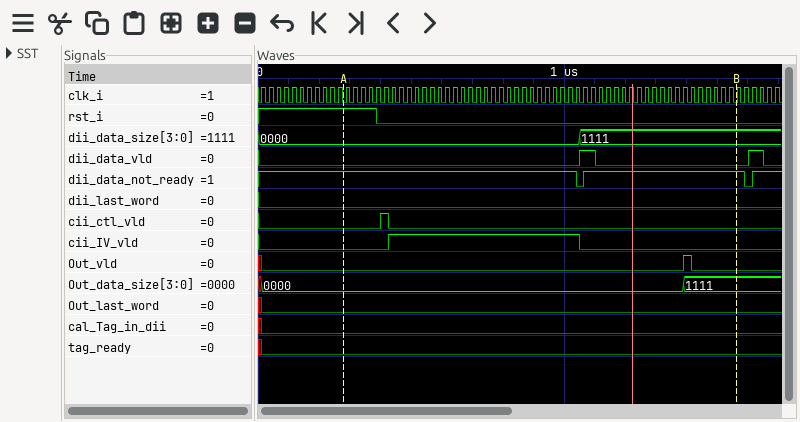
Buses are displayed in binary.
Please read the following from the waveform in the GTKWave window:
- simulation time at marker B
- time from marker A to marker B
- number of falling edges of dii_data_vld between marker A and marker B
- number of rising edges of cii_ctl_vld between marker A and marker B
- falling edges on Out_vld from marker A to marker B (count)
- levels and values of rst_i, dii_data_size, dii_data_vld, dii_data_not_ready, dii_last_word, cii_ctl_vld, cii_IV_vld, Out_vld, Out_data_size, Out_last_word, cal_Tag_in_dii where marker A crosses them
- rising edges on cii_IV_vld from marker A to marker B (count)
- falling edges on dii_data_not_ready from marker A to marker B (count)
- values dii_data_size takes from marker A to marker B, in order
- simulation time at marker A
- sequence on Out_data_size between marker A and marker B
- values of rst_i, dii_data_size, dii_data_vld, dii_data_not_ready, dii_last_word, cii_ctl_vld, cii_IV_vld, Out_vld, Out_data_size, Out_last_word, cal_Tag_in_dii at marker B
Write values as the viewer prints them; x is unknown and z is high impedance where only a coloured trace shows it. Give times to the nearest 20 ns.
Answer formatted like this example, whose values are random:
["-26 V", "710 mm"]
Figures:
["1560 ns", "1280 ns", "1", "1", "1", "rst_i=1, dii_data_size=0000, dii_data_vld=0, dii_data_not_ready=1, dii_last_word=0, cii_ctl_vld=0, cii_IV_vld=0, Out_vld=0, Out_data_size=0000, Out_last_word=0, cal_Tag_in_dii=0", "1", "1", "0000, 1111", "280 ns", "0000, 1111", "rst_i=0, dii_data_size=1111, dii_data_vld=0, dii_data_not_ready=1, dii_last_word=0, cii_ctl_vld=0, cii_IV_vld=0, Out_vld=0, Out_data_size=1111, Out_last_word=0, cal_Tag_in_dii=0"]
